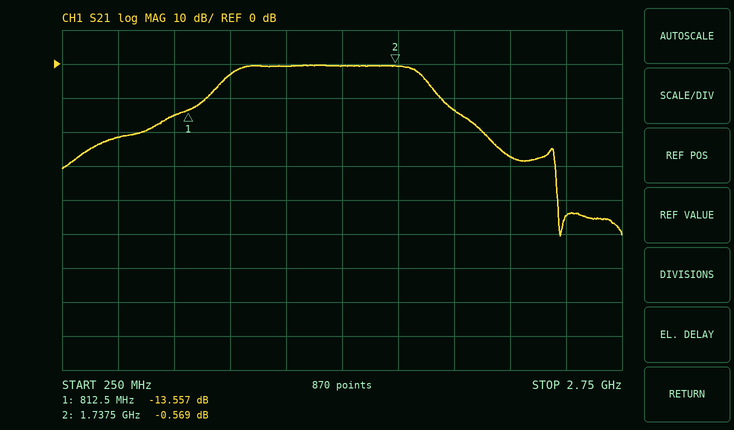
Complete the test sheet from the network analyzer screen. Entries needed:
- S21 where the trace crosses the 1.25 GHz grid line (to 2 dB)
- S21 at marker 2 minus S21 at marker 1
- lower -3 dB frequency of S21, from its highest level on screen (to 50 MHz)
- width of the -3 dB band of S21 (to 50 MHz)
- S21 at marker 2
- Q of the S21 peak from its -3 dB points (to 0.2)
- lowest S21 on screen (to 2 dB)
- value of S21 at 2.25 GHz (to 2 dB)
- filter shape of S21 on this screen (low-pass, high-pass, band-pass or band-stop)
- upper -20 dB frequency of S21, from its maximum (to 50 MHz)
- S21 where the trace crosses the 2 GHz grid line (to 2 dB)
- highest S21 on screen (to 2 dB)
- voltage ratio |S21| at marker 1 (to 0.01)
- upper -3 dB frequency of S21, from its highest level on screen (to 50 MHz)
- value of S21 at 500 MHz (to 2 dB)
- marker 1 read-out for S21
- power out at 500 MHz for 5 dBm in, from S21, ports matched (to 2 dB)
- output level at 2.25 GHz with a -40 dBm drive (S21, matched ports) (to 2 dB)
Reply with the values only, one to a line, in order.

0 dB
12.988 dB
1.00 GHz
850 MHz
-0.569 dB
1.6
-50 dB
-28 dB
band-pass
2.15 GHz
-14 dB
0 dB
0.21
1.85 GHz
-22 dB
-13.557 dB
-16 dBm
-68 dBm
